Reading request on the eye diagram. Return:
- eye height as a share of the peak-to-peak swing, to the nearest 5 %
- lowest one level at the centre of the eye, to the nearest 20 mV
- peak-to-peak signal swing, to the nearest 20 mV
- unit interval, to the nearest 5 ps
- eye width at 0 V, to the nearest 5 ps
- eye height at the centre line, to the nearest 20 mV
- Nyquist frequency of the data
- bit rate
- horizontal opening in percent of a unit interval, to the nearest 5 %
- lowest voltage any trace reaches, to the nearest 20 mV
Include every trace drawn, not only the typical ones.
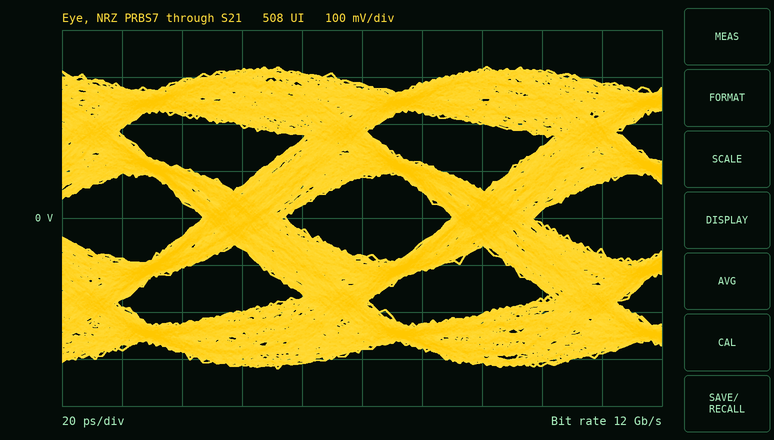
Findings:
25 %
80 mV
640 mV
85 ps
55 ps
160 mV
6 GHz
12 Gb/s
65 %
-320 mV
